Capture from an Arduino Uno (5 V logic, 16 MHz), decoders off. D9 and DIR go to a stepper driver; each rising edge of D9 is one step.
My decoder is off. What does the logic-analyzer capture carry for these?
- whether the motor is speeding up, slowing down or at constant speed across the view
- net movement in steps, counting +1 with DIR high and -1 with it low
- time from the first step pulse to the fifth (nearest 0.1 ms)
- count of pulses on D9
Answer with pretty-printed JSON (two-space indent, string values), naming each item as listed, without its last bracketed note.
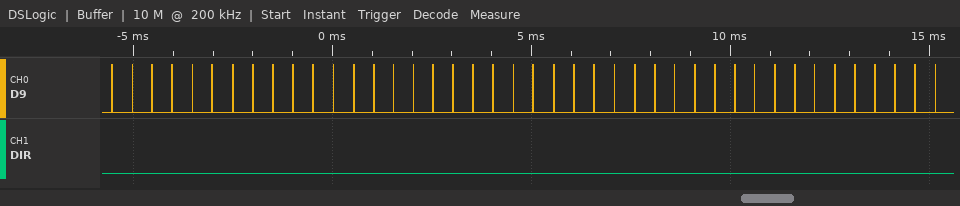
{
  "whether the motor is speeding up, slowing down or at constant speed across the view": "constant speed",
  "net movement in steps, counting +1 with DIR high and -1 with it low": "-42",
  "time from the first step pulse to the fifth": "2.0 ms",
  "count of pulses on D9": "42"
}
